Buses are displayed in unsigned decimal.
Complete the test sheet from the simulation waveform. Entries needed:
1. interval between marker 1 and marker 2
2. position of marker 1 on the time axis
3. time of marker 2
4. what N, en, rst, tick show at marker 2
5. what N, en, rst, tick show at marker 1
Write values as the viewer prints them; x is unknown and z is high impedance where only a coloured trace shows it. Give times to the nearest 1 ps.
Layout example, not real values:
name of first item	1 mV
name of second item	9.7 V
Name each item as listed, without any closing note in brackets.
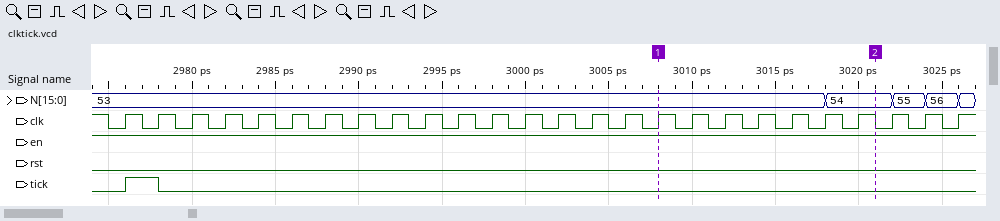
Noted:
interval between marker 1 and marker 2	13 ps
position of marker 1 on the time axis	3008 ps
time of marker 2	3021 ps
what N, en, rst, tick show at marker 2	N=54, en=1, rst=0, tick=0
what N, en, rst, tick show at marker 1	N=53, en=1, rst=0, tick=0
